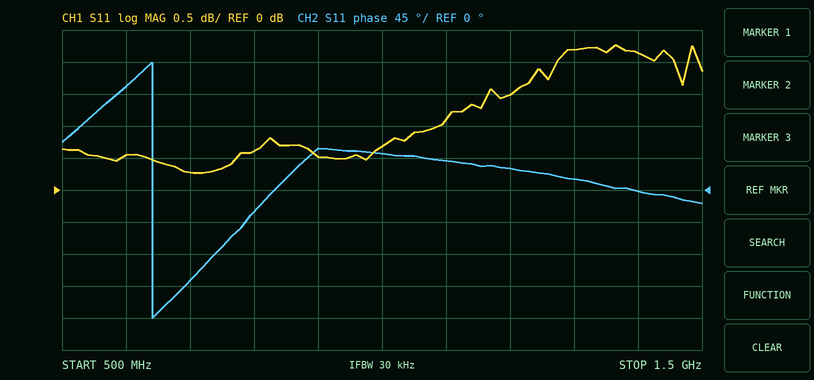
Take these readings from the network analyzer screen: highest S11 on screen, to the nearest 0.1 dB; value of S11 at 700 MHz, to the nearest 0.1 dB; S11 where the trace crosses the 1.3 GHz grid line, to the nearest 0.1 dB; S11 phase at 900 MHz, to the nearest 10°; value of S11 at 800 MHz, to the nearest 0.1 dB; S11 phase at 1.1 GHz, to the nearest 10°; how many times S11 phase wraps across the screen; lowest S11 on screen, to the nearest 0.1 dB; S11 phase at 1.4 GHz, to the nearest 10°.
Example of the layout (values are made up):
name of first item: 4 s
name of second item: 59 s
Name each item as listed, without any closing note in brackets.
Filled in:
highest S11 on screen, to the nearest 0.1 dB: 2.3 dB
value of S11 at 700 MHz, to the nearest 0.1 dB: 0.3 dB
S11 where the trace crosses the 1.3 GHz grid line, to the nearest 0.1 dB: 2.2 dB
S11 phase at 900 MHz, to the nearest 10°: 60°
value of S11 at 800 MHz, to the nearest 0.1 dB: 0.6 dB
S11 phase at 1.1 GHz, to the nearest 10°: 40°
how many times S11 phase wraps across the screen: 1
lowest S11 on screen, to the nearest 0.1 dB: 0.3 dB
S11 phase at 1.4 GHz, to the nearest 10°: 0°
